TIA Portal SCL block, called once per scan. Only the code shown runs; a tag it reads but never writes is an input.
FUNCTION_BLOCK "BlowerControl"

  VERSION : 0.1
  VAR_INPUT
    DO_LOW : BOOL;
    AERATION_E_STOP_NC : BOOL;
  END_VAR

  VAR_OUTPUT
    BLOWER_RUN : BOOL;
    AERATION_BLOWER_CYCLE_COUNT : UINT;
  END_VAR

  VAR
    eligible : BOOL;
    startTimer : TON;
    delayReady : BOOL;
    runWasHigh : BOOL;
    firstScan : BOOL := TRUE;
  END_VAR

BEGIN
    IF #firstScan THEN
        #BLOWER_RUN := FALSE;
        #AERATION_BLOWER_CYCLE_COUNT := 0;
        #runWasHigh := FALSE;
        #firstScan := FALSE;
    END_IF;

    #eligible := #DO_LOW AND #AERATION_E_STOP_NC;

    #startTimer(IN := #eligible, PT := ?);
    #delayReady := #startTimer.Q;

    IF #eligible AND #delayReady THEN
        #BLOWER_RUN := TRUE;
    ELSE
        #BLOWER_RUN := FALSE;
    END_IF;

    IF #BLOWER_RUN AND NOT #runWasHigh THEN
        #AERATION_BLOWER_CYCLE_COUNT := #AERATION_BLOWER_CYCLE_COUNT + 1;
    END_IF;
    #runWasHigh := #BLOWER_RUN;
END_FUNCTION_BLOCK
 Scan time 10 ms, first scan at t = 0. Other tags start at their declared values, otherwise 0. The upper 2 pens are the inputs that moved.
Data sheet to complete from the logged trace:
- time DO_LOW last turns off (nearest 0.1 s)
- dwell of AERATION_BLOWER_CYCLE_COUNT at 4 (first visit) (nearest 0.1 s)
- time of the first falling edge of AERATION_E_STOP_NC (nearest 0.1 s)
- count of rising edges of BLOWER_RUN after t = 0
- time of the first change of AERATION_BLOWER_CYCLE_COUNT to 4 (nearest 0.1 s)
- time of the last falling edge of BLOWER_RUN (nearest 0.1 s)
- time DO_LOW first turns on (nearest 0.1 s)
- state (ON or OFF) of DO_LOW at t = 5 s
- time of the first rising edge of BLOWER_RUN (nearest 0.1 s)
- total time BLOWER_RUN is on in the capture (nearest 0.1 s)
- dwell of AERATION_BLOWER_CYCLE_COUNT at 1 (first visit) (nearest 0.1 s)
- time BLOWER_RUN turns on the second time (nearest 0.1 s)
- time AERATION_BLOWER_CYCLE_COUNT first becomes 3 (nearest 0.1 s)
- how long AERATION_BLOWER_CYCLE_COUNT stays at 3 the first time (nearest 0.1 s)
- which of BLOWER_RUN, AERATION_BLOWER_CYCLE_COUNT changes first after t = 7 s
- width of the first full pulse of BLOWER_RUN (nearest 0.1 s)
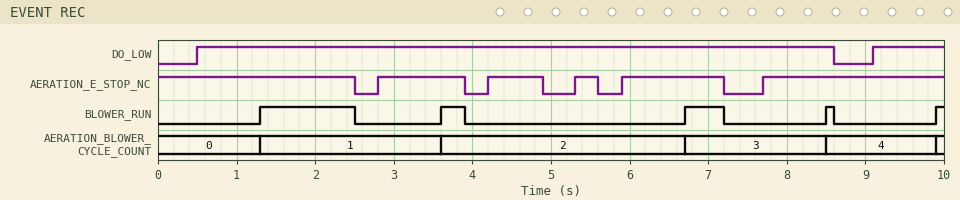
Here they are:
8.6 s
1.4 s
2.5 s
5
8.5 s
8.6 s
0.5 s
ON
1.3 s
2.2 s
2.3 s
3.6 s
6.7 s
1.8 s
BLOWER_RUN
1.2 s
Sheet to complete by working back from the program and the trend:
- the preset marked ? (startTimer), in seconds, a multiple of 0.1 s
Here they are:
0.8 s
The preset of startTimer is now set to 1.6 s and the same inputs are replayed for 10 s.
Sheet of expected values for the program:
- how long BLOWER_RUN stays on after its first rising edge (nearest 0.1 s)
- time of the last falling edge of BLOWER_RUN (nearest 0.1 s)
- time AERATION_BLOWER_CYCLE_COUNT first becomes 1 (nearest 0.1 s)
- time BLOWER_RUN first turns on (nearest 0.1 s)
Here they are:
0.4 s
2.5 s
2.1 s
2.1 s
